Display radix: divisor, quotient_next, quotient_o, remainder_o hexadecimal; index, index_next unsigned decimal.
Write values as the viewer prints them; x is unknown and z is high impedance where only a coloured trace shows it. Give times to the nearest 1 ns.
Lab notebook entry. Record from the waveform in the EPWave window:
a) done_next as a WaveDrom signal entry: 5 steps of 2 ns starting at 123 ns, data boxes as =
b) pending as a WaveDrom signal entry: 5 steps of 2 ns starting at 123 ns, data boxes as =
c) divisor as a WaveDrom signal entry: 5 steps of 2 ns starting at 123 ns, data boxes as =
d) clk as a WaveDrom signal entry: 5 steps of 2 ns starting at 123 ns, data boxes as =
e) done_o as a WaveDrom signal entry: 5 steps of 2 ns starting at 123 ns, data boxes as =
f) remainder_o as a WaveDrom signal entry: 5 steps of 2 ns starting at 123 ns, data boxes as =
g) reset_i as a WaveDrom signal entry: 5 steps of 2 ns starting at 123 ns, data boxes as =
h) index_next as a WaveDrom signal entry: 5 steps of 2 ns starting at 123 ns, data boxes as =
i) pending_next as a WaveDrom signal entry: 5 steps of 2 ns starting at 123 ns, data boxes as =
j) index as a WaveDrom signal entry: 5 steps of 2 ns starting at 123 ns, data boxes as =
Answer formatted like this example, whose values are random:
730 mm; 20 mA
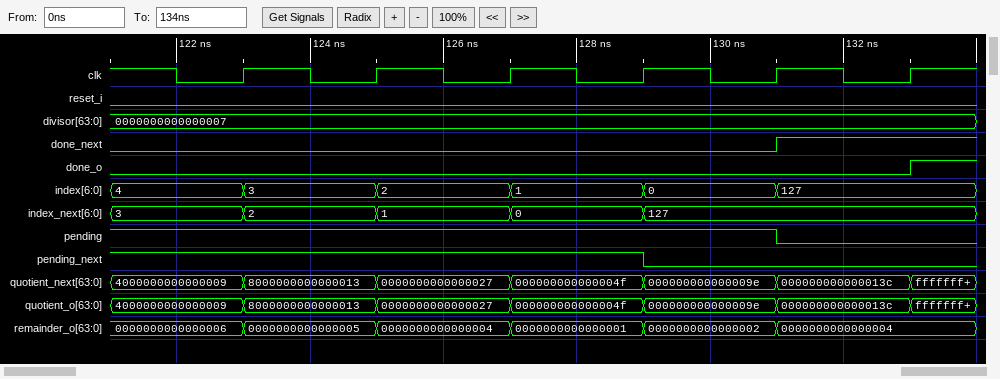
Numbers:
{name: 'done_next', wave: '0...1'}; {name: 'pending', wave: '1...0'}; {name: 'divisor', wave: '=....', data: '0000000000000007'}; {name: 'clk', wave: 'p....'}; {name: 'done_o', wave: '0....'}; {name: 'remainder_o', wave: '=====', data: '0000000000000005 0000000000000004 0000000000000001 0000000000000002 0000000000000004'}; {name: 'reset_i', wave: '0....'}; {name: 'index_next', wave: '====.', data: '2 1 0 127'}; {name: 'pending_next', wave: '1..0.'}; {name: 'index', wave: '=====', data: '3 2 1 0 127'}
